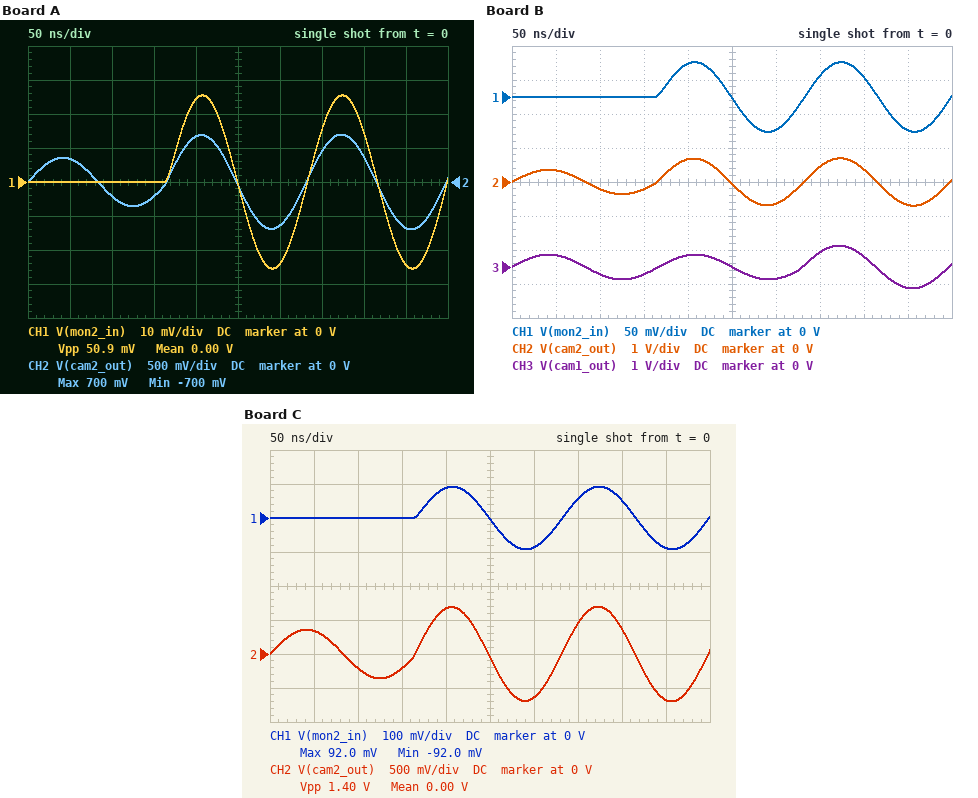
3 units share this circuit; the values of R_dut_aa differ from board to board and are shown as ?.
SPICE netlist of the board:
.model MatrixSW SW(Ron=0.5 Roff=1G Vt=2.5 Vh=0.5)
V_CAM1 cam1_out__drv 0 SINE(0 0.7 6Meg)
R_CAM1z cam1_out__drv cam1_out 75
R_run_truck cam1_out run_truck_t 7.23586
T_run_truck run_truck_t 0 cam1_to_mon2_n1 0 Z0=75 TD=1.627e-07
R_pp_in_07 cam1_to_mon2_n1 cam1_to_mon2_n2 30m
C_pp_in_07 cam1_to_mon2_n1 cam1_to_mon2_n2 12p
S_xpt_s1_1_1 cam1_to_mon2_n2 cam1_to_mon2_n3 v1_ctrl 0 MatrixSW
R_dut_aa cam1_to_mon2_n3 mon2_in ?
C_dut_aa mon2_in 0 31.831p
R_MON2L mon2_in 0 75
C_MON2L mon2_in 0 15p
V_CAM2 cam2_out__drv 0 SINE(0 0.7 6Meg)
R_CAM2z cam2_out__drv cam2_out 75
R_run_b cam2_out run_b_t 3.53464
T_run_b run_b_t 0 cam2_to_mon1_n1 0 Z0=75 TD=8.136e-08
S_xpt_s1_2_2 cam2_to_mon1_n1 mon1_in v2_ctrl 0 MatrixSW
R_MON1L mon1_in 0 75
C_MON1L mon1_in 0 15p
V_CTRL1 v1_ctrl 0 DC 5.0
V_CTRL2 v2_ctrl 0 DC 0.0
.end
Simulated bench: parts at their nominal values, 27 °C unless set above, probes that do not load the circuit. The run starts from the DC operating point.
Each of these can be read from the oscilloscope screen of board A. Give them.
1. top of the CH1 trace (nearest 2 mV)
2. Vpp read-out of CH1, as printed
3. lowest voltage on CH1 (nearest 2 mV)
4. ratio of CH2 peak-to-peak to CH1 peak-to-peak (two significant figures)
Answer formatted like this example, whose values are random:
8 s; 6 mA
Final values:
26 mV; 50.9 mV; -26 mV; 27
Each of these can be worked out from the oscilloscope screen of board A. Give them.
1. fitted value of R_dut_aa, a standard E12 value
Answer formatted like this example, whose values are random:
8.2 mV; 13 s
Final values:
1.8 kΩ
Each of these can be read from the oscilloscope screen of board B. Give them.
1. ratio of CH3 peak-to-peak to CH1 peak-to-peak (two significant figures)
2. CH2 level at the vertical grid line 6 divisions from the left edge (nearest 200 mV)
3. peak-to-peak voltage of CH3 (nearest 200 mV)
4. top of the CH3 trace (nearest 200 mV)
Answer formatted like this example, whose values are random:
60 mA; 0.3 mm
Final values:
12; -600 mV; 1.2 V; 600 mV
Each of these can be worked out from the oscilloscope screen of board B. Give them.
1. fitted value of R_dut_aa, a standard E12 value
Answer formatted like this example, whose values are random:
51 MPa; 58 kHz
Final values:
820 Ω
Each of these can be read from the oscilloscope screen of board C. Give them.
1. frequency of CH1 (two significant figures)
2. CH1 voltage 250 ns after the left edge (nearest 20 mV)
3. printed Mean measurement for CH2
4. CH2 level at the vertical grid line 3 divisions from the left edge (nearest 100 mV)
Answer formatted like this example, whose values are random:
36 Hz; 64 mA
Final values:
6.0 MHz; 0 V; 0.00 V; -200 mV
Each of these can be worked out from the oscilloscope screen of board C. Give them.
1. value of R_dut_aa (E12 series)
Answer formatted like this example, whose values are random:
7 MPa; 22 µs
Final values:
390 Ω
